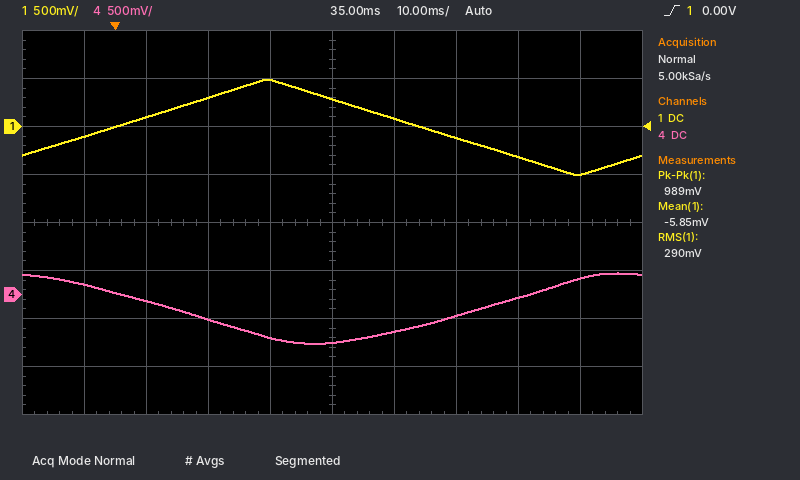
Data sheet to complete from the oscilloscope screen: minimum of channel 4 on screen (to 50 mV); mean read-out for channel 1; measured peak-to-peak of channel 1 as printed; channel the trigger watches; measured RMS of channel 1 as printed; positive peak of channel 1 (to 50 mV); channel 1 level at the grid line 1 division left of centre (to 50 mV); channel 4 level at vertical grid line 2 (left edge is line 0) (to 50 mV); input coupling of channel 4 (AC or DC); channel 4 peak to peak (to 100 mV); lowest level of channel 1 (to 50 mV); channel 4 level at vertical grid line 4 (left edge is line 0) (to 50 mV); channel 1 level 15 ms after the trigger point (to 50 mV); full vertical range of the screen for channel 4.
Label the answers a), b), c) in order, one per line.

a) -500 mV
b) -5.85 mV
c) 989 mV
d) channel 1
e) 290 mV
f) 500 mV
g) 500 mV
h) -50 mV
i) DC
j) 700 mV
k) -500 mV
l) -450 mV
m) 300 mV
n) 4 V
